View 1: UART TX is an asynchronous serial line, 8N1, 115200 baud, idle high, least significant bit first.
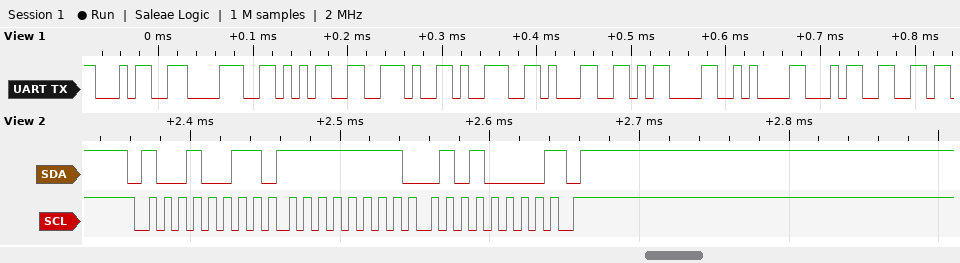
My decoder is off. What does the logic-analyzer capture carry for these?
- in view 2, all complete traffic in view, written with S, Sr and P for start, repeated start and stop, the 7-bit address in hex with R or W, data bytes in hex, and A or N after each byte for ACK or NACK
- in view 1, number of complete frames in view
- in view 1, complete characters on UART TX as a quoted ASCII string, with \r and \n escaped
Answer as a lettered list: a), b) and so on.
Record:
a) S 49R A FF A 50 N P
b) 9
c) "485.91\r\n4"
